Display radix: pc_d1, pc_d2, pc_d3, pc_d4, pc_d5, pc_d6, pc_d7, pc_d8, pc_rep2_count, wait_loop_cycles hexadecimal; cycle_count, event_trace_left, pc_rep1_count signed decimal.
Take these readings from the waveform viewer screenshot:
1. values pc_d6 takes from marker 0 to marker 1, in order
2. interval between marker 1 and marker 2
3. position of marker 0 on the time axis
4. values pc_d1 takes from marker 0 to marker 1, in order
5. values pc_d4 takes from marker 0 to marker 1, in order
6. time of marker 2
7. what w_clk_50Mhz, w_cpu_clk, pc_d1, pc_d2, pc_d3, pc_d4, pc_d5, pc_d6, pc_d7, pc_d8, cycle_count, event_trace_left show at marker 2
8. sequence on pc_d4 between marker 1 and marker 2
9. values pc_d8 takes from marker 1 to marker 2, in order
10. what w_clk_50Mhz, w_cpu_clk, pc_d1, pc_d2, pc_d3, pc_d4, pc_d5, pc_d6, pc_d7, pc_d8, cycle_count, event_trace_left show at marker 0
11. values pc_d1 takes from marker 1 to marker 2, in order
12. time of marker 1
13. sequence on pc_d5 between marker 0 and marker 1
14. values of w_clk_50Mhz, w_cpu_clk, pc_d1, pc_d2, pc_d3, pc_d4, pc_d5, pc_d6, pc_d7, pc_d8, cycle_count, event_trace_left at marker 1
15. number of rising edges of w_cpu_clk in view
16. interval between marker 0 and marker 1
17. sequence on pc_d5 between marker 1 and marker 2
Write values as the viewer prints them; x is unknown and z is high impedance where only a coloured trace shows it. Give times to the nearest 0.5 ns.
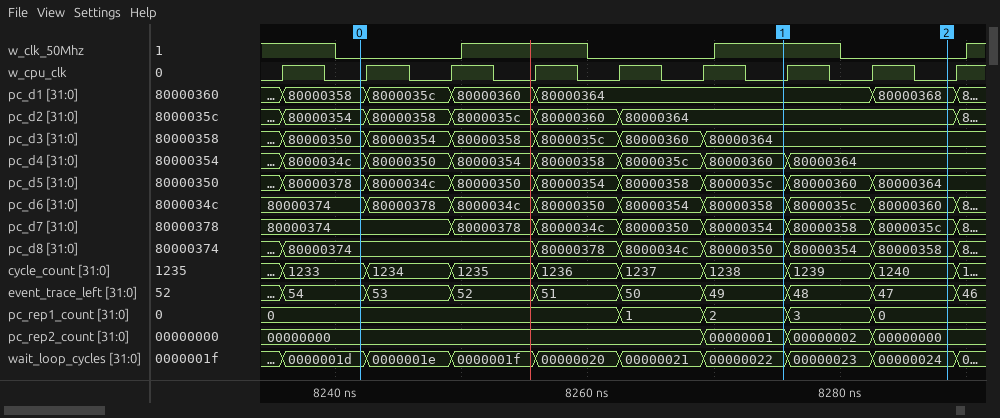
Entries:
80000374, 80000378, 8000034c, 80000350, 80000354, 80000358
13 ns
8242 ns
80000358, 8000035c, 80000360, 80000364
8000034c, 80000350, 80000354, 80000358, 8000035c, 80000360
8288.5 ns
w_clk_50Mhz=0, w_cpu_clk=0, pc_d1=80000368, pc_d2=80000364, pc_d3=80000364, pc_d4=80000364, pc_d5=80000364, pc_d6=80000360, pc_d7=8000035c, pc_d8=80000358, cycle_count=1240, event_trace_left=47
80000360, 80000364
80000350, 80000354, 80000358
w_clk_50Mhz=0, w_cpu_clk=0, pc_d1=80000358, pc_d2=80000354, pc_d3=80000350, pc_d4=8000034c, pc_d5=80000378, pc_d6=80000374, pc_d7=80000374, pc_d8=80000374, cycle_count=1233, event_trace_left=54
80000364, 80000368
8275.5 ns
80000378, 8000034c, 80000350, 80000354, 80000358, 8000035c
w_clk_50Mhz=1, w_cpu_clk=0, pc_d1=80000364, pc_d2=80000364, pc_d3=80000364, pc_d4=80000360, pc_d5=8000035c, pc_d6=80000358, pc_d7=80000354, pc_d8=80000350, cycle_count=1238, event_trace_left=49
9
33.5 ns
8000035c, 80000360, 80000364
